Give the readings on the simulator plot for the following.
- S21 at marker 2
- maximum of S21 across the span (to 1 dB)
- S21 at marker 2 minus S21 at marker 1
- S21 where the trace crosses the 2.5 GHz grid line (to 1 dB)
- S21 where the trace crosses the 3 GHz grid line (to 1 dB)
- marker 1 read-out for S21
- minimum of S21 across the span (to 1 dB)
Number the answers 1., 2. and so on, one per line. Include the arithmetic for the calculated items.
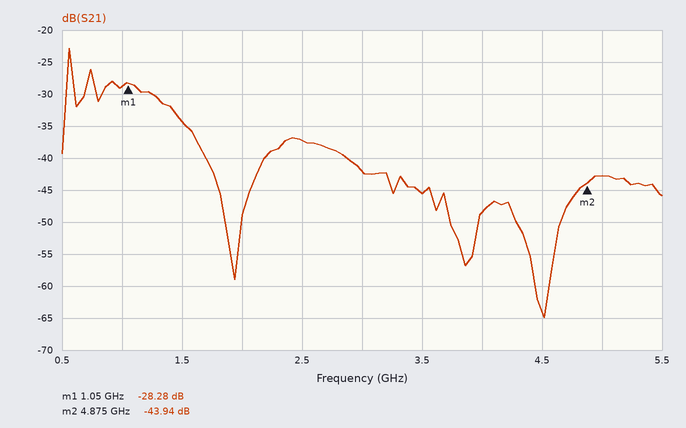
1. -43.94 dB
2. -23 dB
3. -43.94 − (-28.28) = -15.66 dB
4. -37 dB
5. -42 dB
6. -28.28 dB
7. -65 dB
